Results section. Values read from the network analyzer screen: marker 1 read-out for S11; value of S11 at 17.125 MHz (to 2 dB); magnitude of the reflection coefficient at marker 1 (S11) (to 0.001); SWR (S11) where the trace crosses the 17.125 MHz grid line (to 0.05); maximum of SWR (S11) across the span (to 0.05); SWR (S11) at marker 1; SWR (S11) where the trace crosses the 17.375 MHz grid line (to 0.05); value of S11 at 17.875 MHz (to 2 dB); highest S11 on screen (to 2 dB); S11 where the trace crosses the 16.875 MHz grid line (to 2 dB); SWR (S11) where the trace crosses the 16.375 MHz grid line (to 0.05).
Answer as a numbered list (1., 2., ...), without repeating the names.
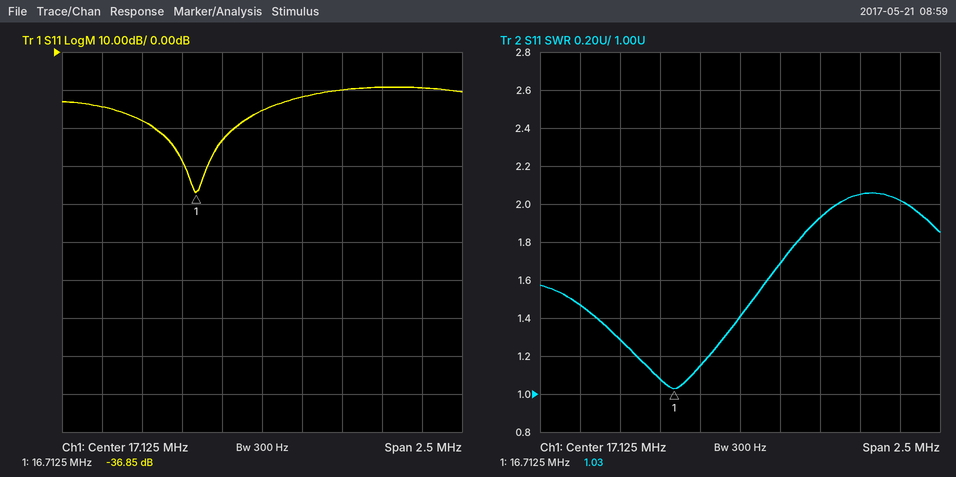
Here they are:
1. -36.85 dB
2. -16 dB
3. 0.014
4. 1.40
5. 2.05
6. 1.03
7. 1.70
8. -10 dB
9. -10 dB
10. -24 dB
11. 1.30
